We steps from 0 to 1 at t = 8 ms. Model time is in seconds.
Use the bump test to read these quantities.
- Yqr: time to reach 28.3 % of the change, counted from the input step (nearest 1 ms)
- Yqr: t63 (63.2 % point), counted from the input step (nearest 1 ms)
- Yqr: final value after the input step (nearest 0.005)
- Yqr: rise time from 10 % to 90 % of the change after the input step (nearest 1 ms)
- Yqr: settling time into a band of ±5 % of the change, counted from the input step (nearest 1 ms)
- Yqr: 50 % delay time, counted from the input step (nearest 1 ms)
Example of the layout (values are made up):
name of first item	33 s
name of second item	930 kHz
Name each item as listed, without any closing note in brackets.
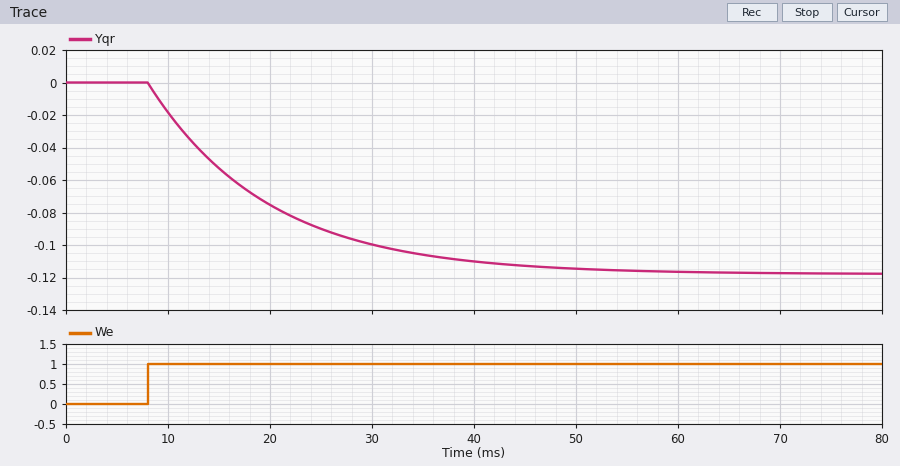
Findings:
Yqr: time to reach 28.3 % of the change, counted from the input step	4 ms
Yqr: t63 (63.2 % point), counted from the input step	12 ms
Yqr: final value after the input step	-0.120
Yqr: rise time from 10 % to 90 % of the change after the input step	26 ms
Yqr: settling time into a band of ±5 % of the change, counted from the input step	35 ms
Yqr: 50 % delay time, counted from the input step	8 ms
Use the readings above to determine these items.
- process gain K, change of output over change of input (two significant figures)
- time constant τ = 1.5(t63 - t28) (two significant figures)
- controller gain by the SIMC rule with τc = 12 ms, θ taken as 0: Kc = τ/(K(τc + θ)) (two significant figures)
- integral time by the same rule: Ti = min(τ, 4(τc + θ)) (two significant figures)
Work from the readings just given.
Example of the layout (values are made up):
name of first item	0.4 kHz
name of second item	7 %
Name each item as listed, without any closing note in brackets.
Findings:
process gain K, change of output over change of input	-0.12
time constant τ = 1.5(t63 - t28)	12 ms
controller gain by the SIMC rule with τc = 12 ms, θ taken as 0: Kc = τ/(K(τc + θ))	-8.3
integral time by the same rule: Ti = min(τ, 4(τc + θ))	12 ms
